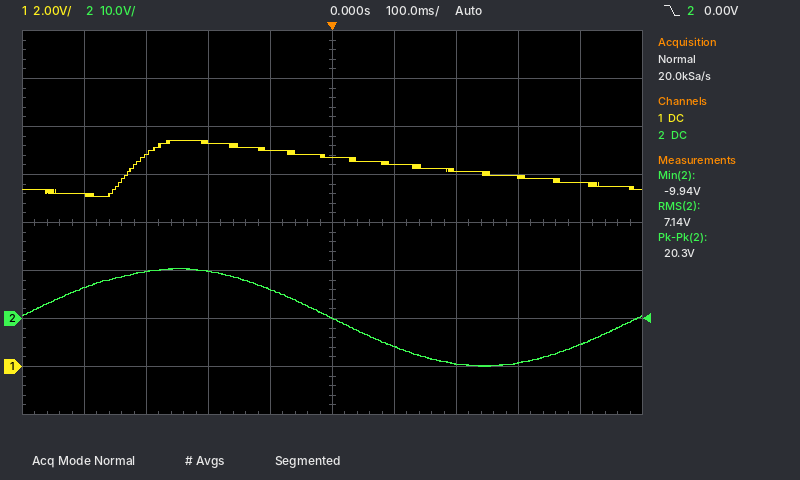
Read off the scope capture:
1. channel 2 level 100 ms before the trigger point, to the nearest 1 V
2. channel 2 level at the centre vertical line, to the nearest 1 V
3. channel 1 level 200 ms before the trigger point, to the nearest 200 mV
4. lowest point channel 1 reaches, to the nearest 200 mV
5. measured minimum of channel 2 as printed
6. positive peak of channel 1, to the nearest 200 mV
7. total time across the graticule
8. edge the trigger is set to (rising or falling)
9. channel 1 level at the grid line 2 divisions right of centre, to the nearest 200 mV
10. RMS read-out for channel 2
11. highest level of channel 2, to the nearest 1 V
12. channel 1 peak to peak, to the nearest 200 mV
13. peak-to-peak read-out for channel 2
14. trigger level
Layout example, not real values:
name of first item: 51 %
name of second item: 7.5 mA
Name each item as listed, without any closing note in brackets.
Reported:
channel 2 level 100 ms before the trigger point, to the nearest 1 V: 6 V
channel 2 level at the centre vertical line, to the nearest 1 V: 0 V
channel 1 level 200 ms before the trigger point, to the nearest 200 mV: 9.4 V
lowest point channel 1 reaches, to the nearest 200 mV: 7.0 V
measured minimum of channel 2 as printed: -9.94 V
positive peak of channel 1, to the nearest 200 mV: 9.4 V
total time across the graticule: 1 s
edge the trigger is set to: falling
channel 1 level at the grid line 2 divisions right of centre, to the nearest 200 mV: 8.2 V
RMS read-out for channel 2: 7.14 V
highest level of channel 2, to the nearest 1 V: 10 V
channel 1 peak to peak, to the nearest 200 mV: 2.4 V
peak-to-peak read-out for channel 2: 20.3 V
trigger level: 0.00 V
